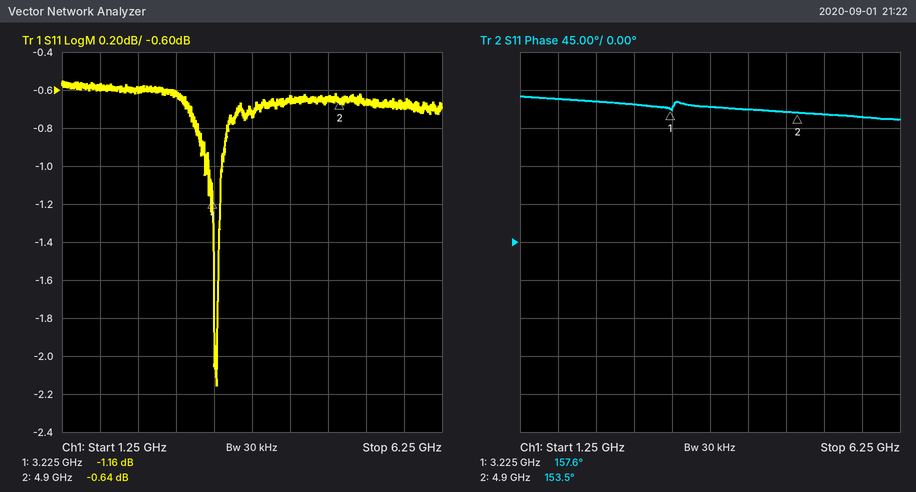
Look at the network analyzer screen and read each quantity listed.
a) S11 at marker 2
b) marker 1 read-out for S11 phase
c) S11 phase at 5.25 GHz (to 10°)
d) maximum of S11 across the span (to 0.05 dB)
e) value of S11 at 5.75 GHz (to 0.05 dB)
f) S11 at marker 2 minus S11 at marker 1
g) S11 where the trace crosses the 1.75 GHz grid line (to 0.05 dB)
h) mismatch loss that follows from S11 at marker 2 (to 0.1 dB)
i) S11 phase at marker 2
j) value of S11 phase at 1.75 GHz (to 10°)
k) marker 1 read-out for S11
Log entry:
-0.64 dB
157.6°
150°
-0.55 dB
-0.70 dB
0.52 dB
-0.60 dB
8.6 dB
153.5°
170°
-1.16 dB
